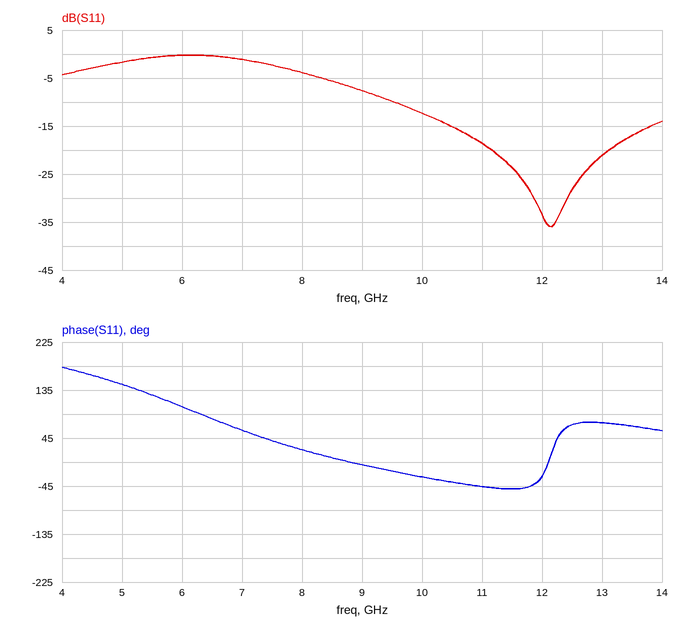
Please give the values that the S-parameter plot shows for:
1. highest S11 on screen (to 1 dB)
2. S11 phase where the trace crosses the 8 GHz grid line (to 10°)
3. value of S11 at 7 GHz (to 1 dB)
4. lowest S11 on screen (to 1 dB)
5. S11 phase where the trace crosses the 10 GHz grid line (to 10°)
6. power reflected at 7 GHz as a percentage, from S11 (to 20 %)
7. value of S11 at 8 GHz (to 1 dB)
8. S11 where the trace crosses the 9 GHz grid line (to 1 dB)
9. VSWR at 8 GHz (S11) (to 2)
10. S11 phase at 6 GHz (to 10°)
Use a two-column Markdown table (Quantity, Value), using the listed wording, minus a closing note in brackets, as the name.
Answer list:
| Quantity | Value |
|---|---|
| highest S11 on screen | 0 dB |
| S11 phase where the trace crosses the 8 GHz grid line | 20° |
| value of S11 at 7 GHz | -1 dB |
| lowest S11 on screen | -36 dB |
| S11 phase where the trace crosses the 10 GHz grid line | -30° |
| power reflected at 7 GHz as a percentage, from S11 | 80 % |
| value of S11 at 8 GHz | -4 dB |
| S11 where the trace crosses the 9 GHz grid line | -8 dB |
| VSWR at 8 GHz (S11) | 4 |
| S11 phase at 6 GHz | 100° |
